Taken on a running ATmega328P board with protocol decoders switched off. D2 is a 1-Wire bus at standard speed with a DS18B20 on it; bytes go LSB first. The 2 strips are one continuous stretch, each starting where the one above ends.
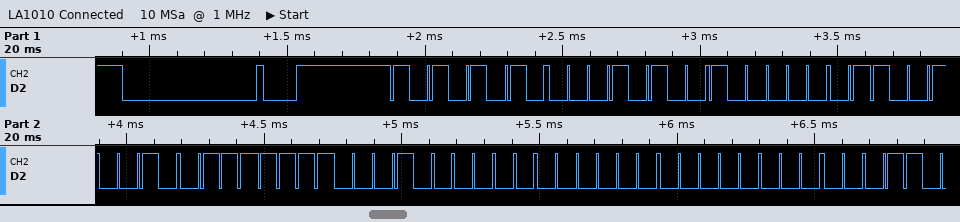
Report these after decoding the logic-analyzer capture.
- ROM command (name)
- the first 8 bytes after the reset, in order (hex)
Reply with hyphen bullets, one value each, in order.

- Match ROM
- 55 28 81 49 FE 08 00 00
